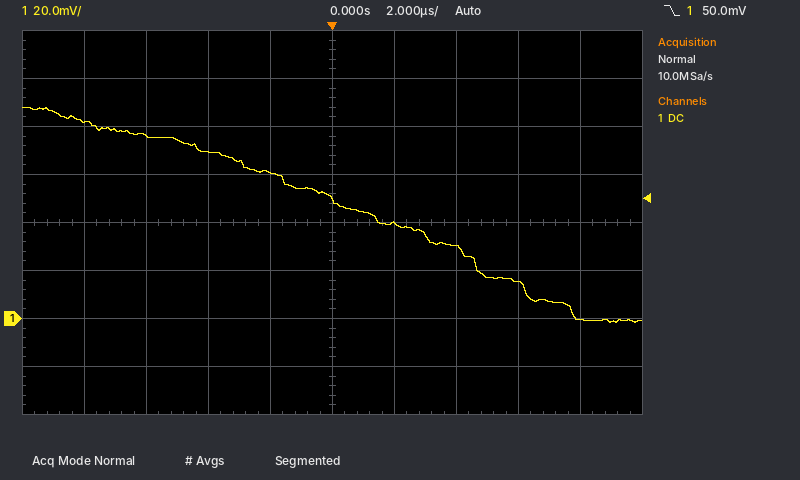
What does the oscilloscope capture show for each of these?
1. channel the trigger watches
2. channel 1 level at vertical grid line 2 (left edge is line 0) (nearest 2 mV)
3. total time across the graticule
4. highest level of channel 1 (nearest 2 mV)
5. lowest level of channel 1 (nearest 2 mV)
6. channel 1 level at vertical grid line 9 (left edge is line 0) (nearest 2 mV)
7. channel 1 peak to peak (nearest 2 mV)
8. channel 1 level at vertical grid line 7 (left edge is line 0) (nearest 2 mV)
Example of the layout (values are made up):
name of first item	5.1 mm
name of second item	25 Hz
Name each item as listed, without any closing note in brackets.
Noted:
channel the trigger watches	channel 1
channel 1 level at vertical grid line 2 (left edge is line 0)	76 mV
total time across the graticule	20 µs
highest level of channel 1	88 mV
lowest level of channel 1	-2 mV
channel 1 level at vertical grid line 9 (left edge is line 0)	0 mV
channel 1 peak to peak	90 mV
channel 1 level at vertical grid line 7 (left edge is line 0)	30 mV
